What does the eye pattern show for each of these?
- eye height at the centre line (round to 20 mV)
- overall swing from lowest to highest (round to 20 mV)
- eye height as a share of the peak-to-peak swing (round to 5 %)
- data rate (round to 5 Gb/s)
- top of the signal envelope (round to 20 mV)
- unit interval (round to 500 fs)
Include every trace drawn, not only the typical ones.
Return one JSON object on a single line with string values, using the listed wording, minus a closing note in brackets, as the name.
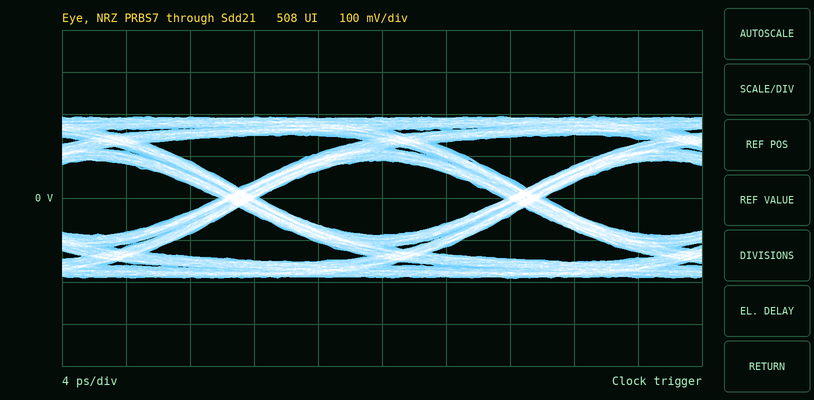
{"eye height at the centre line": "180 mV", "overall swing from lowest to highest": "380 mV", "eye height as a share of the peak-to-peak swing": "45 %", "data rate": "55 Gb/s", "top of the signal envelope": "200 mV", "unit interval": "18.0 ps"}
